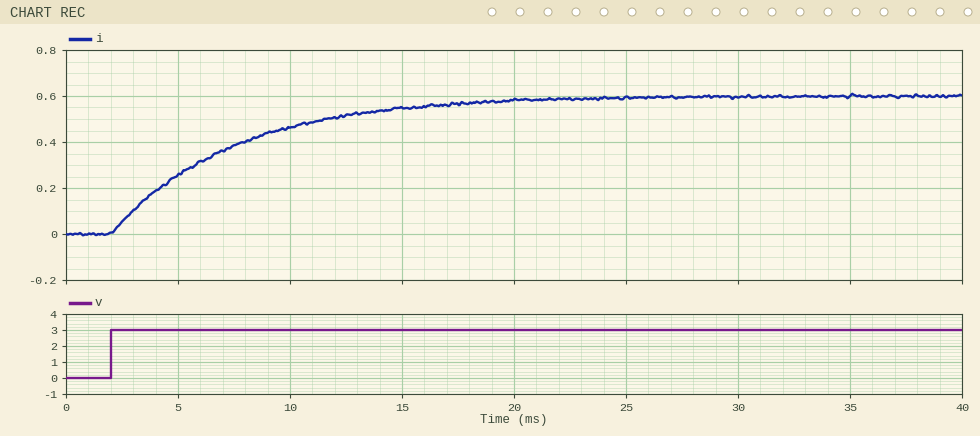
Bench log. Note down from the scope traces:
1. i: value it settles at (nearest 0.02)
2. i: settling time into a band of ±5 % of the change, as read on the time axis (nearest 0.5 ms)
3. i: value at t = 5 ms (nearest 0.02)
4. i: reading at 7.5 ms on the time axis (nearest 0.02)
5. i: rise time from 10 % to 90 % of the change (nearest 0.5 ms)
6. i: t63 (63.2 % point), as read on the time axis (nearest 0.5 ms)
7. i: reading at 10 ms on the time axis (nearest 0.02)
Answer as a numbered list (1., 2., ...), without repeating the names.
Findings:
1. 0.60
2. 18.0 ms
3. 0.26
4. 0.38
5. 12.0 ms
6. 7.5 ms
7. 0.46
